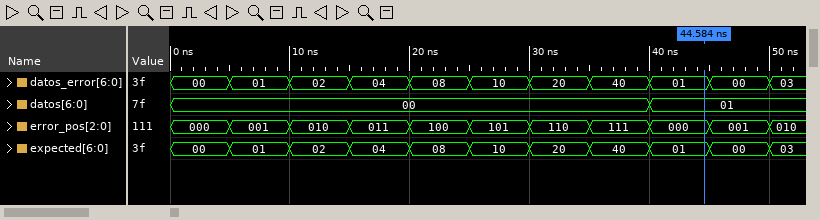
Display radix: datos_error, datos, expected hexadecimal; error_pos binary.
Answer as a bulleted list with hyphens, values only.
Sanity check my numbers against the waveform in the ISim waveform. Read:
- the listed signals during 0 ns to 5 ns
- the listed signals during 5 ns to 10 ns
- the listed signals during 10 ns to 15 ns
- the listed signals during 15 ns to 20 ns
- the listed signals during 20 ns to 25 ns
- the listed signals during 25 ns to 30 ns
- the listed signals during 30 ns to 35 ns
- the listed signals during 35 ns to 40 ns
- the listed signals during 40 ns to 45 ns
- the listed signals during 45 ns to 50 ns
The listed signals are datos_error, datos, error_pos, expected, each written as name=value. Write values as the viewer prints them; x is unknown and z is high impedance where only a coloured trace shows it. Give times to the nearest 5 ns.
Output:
- datos_error=00, datos=00, error_pos=000, expected=00
- datos_error=01, datos=00, error_pos=001, expected=01
- datos_error=02, datos=00, error_pos=010, expected=02
- datos_error=04, datos=00, error_pos=011, expected=04
- datos_error=08, datos=00, error_pos=100, expected=08
- datos_error=10, datos=00, error_pos=101, expected=10
- datos_error=20, datos=00, error_pos=110, expected=20
- datos_error=40, datos=00, error_pos=111, expected=40
- datos_error=01, datos=01, error_pos=000, expected=01
- datos_error=00, datos=01, error_pos=001, expected=00
